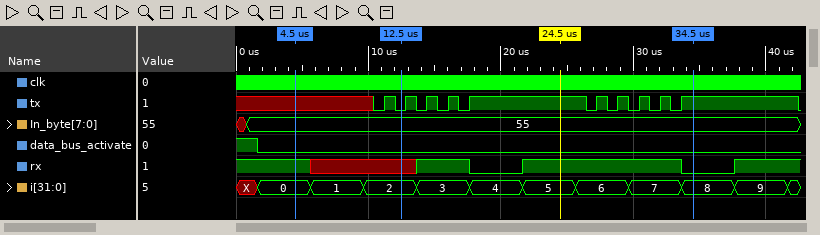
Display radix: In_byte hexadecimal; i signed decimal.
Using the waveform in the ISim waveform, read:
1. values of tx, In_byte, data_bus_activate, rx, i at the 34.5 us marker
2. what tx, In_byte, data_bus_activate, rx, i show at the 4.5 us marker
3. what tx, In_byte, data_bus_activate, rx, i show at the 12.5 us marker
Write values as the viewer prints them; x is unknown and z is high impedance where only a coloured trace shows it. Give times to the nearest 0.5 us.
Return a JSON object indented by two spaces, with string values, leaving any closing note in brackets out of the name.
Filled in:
{
  "values of tx, In_byte, data_bus_activate, rx, i at the 34.5 us marker": "tx=1, In_byte=55, data_bus_activate=0, rx=0, i=8",
  "what tx, In_byte, data_bus_activate, rx, i show at the 4.5 us marker": "tx=x, In_byte=55, data_bus_activate=0, rx=1, i=0",
  "what tx, In_byte, data_bus_activate, rx, i show at the 12.5 us marker": "tx=0, In_byte=55, data_bus_activate=0, rx=x, i=2"
}
